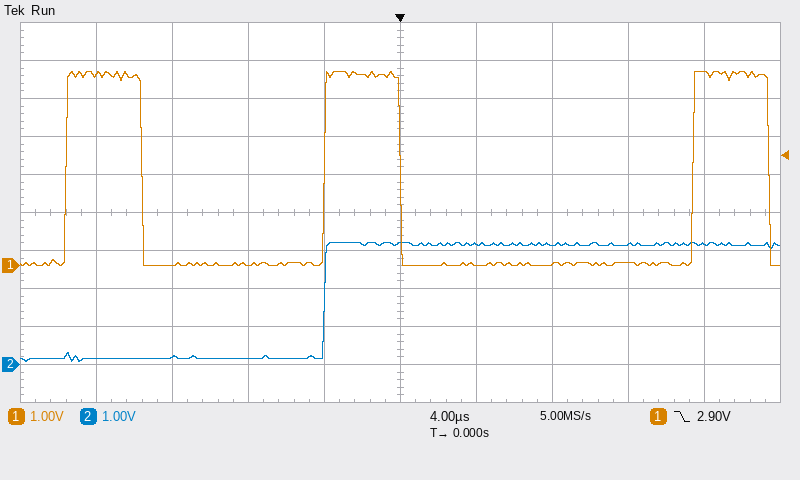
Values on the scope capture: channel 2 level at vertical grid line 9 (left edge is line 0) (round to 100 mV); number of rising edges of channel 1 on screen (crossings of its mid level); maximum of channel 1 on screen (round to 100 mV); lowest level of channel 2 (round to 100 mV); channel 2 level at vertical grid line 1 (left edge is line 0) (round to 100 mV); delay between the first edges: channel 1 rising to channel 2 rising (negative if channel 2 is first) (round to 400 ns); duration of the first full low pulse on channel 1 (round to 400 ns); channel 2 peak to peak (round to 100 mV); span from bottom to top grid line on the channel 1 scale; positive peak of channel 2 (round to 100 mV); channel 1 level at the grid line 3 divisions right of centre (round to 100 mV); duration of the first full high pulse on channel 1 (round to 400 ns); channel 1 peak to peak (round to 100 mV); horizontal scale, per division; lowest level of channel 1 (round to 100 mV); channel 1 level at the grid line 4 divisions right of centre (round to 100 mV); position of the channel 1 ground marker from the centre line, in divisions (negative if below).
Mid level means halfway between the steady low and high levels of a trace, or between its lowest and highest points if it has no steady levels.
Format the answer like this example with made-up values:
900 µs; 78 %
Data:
3.2 V; 3; 5.1 V; 100 mV; 200 mV; +13.6 µs; 9.6 µs; 3.1 V; 10 V; 3.2 V; 100 mV; 4.0 µs; 5.1 V; 4 µs; 0.0 V; 5.1 V; -1.4 div
